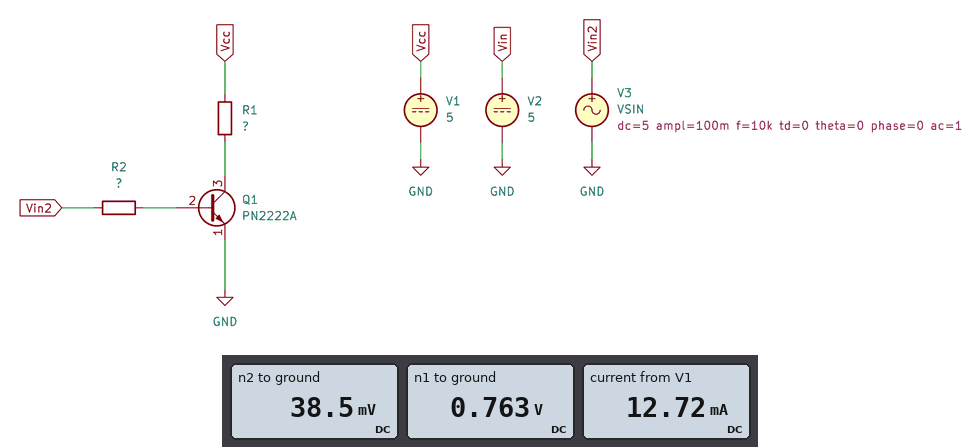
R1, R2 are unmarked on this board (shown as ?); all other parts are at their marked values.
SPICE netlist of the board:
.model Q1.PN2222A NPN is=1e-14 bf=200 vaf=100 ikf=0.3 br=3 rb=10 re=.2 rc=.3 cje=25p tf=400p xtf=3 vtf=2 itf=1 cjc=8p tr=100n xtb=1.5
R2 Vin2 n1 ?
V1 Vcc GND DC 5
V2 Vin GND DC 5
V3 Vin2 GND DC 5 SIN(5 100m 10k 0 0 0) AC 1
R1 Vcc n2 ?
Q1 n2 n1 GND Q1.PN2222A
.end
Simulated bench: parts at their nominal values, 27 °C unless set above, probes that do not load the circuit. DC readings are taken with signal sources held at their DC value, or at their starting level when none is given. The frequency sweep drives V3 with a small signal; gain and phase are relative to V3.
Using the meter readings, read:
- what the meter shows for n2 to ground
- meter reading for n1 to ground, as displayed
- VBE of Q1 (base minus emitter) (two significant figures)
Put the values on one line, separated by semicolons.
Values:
38.5 mV; 0.763 V; 760 mV
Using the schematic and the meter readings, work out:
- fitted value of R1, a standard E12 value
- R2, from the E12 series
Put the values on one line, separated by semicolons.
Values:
390 Ω; 1.8 kΩ
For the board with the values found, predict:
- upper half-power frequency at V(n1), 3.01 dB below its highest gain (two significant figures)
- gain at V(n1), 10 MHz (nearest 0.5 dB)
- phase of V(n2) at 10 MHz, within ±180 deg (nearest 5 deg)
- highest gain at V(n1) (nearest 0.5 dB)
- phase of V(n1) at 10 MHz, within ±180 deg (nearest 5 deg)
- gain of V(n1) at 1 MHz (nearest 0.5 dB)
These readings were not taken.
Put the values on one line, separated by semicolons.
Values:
600 MHz; -44.0 dB; 15 deg; -41.5 dB; 0 deg; -43.5 dB
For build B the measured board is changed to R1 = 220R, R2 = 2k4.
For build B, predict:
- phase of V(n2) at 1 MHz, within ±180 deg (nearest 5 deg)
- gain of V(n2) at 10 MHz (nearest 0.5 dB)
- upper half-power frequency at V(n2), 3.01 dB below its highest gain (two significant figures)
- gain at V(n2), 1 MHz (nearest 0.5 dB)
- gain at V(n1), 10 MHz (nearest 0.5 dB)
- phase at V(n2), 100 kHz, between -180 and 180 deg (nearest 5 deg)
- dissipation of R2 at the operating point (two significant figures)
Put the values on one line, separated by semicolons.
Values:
110 deg; -65.0 dB; 540 kHz; -52.5 dB; -46.5 dB; 170 deg; 7.5 mW
